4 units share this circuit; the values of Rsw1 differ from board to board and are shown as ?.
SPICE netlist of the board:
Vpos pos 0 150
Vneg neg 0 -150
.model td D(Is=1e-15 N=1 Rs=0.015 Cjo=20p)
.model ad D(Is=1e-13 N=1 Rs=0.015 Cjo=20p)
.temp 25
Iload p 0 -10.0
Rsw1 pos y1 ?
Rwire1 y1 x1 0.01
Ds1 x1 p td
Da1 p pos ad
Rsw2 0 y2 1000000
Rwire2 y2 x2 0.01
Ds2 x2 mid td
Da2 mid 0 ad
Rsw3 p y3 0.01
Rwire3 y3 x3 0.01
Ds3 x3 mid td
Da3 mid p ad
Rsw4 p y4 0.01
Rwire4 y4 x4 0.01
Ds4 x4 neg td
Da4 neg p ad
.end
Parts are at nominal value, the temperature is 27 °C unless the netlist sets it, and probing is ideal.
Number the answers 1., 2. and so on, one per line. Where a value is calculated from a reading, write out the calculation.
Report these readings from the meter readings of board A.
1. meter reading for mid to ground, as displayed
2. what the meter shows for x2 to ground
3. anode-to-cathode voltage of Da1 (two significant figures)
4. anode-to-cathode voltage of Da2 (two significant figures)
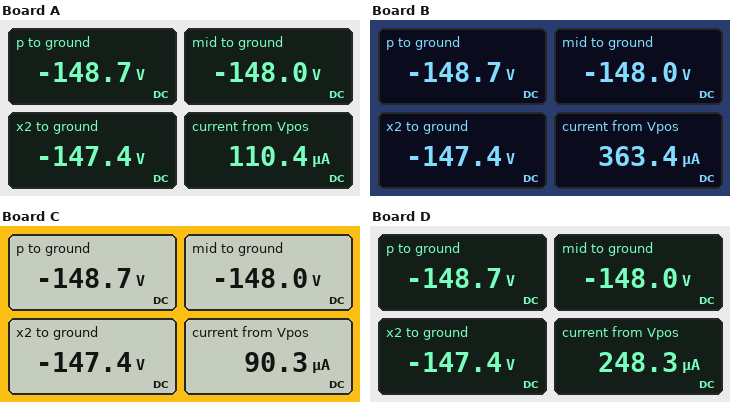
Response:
1. -148.0 V
2. -147.4 V
3. -148.7 V - 150 V = -300 V
4. -148 V = -150 V
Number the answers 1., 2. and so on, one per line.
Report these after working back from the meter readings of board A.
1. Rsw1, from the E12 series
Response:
1. 2.7 MΩ
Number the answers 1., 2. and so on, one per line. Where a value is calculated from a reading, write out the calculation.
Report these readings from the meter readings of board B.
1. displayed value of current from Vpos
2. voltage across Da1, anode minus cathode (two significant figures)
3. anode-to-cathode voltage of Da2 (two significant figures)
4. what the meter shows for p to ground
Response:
1. 363.4 µA
2. -148.7 V - 150 V = -300 V
3. -148 V = -150 V
4. -148.7 V
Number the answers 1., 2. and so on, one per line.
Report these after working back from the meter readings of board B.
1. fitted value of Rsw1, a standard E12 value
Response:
1. 820 kΩ
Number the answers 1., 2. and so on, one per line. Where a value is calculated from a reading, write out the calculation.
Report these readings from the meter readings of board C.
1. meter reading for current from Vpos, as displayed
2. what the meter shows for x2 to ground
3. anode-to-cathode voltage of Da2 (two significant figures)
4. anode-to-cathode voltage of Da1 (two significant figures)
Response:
1. 90.3 µA
2. -147.4 V
3. -148 V = -150 V
4. -148.7 V - 150 V = -300 V
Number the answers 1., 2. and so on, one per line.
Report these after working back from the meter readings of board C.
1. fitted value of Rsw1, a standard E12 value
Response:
1. 3.3 MΩ
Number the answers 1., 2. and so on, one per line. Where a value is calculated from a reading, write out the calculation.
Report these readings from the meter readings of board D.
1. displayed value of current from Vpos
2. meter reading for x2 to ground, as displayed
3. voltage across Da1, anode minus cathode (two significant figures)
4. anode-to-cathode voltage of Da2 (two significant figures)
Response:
1. 248.3 µA
2. -147.4 V
3. -148.7 V - 150 V = -300 V
4. -148 V = -150 V
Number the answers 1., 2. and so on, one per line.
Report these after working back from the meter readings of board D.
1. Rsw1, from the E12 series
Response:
1. 1.2 MΩ
